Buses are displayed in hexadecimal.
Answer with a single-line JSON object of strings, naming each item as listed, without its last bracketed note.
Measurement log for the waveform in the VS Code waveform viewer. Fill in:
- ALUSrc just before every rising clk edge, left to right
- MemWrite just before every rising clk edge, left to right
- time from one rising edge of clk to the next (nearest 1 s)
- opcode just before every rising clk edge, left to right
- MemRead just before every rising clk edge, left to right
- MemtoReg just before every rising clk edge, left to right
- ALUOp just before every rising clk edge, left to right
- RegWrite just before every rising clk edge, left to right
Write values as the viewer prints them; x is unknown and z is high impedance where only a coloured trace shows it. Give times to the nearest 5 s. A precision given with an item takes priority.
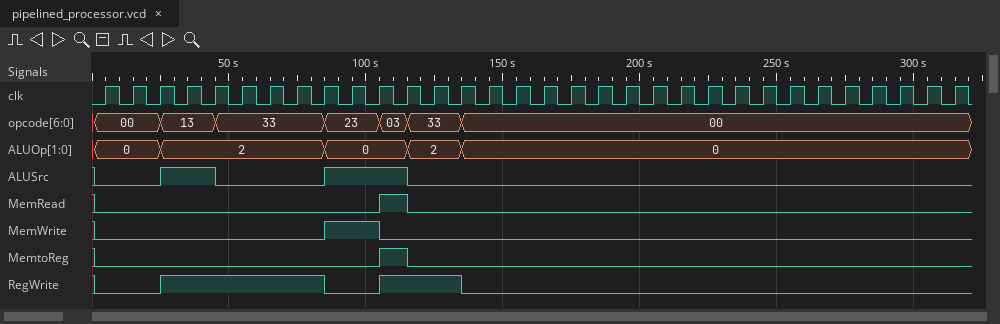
{"ALUSrc just before every rising clk edge, left to right": "0 0 0 1 1 0 0 0 0 1 1 1 0 0 0 0 0 0 0 0 0 0 0 0 0 0 0 0 0 0 0 0", "MemWrite just before every rising clk edge, left to right": "0 0 0 0 0 0 0 0 0 1 1 0 0 0 0 0 0 0 0 0 0 0 0 0 0 0 0 0 0 0 0 0", "time from one rising edge of clk to the next": "10 s", "opcode just before every rising clk edge, left to right": "00, 00, 00, 13, 13, 33, 33, 33, 33, 23, 23, 03, 33, 33, 00, 00, 00, 00, 00, 00, 00, 00, 00, 00, 00, 00, 00, 00, 00, 00, 00, 00", "MemRead just before every rising clk edge, left to right": "0 0 0 0 0 0 0 0 0 0 0 1 0 0 0 0 0 0 0 0 0 0 0 0 0 0 0 0 0 0 0 0", "MemtoReg just before every rising clk edge, left to right": "0 0 0 0 0 0 0 0 0 0 0 1 0 0 0 0 0 0 0 0 0 0 0 0 0 0 0 0 0 0 0 0", "ALUOp just before every rising clk edge, left to right": "0, 0, 0, 2, 2, 2, 2, 2, 2, 0, 0, 0, 2, 2, 0, 0, 0, 0, 0, 0, 0, 0, 0, 0, 0, 0, 0, 0, 0, 0, 0, 0", "RegWrite just before every rising clk edge, left to right": "0 0 0 1 1 1 1 1 1 0 0 1 1 1 0 0 0 0 0 0 0 0 0 0 0 0 0 0 0 0 0 0"}
